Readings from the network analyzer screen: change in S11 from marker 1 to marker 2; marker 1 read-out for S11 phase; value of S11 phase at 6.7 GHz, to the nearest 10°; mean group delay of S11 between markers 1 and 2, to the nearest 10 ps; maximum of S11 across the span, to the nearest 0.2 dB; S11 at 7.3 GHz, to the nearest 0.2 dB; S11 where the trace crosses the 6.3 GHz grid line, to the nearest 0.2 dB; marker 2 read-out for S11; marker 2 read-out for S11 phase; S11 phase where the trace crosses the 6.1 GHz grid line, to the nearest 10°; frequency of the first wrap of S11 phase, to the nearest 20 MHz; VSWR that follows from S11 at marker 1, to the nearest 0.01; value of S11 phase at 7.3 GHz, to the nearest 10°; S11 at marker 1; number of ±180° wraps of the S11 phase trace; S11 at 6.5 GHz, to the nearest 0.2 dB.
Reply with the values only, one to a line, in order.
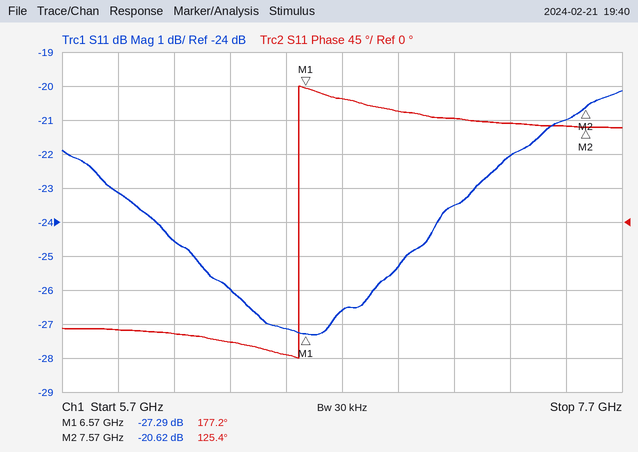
6.67 dB
177.2°
160°
140 ps
-20.2 dB
-22.0 dB
-26.0 dB
-20.62 dB
125.4°
-150°
6.54 GHz
1.09
130°
-27.29 dB
1
-27.2 dB
